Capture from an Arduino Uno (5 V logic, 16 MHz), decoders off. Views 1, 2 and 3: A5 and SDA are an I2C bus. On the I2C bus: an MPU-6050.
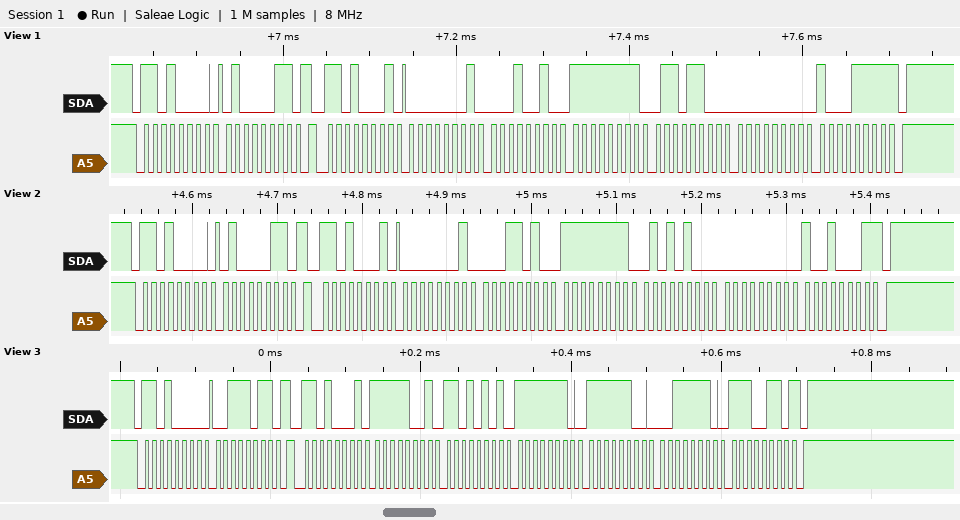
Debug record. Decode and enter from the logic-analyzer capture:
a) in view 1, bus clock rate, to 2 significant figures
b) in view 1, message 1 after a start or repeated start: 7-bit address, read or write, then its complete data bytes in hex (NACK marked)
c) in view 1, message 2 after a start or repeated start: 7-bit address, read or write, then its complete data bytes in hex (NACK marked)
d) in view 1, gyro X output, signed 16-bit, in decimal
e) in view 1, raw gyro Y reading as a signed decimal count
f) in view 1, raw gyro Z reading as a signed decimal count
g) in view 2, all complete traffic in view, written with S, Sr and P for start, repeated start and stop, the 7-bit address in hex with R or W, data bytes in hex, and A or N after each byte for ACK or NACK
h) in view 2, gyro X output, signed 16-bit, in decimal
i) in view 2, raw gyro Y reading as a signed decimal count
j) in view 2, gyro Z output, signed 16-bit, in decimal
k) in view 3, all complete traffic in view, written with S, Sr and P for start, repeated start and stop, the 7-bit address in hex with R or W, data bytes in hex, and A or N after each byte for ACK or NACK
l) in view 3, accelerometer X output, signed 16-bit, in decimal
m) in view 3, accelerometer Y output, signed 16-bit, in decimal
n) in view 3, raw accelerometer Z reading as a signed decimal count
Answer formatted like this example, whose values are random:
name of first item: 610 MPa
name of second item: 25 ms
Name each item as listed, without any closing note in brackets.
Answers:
in view 1, bus clock rate, to 2 significant figures: 100 kHz
in view 1, message 1 after a start or repeated start: 7-bit address, read or write, then its complete data bytes in hex: 0x68 write: 43
in view 1, message 2 after a start or repeated start: 7-bit address, read or write, then its complete data bytes in hex: 0x68 read: 01 12 FF 6C 00 8F NACK
in view 1, gyro X output, signed 16-bit, in decimal: 274
in view 1, raw gyro Y reading as a signed decimal count: -148
in view 1, raw gyro Z reading as a signed decimal count: 143
in view 2, all complete traffic in view, written with S, Sr and P for start, repeated start and stop, the 7-bit address in hex with R or W, data bytes in hex, and A or N after each byte for ACK or NACK: S 68W A 43 A Sr 68R A 01 A 1A A FF A 54 A 00 A 91 N P
in view 2, gyro X output, signed 16-bit, in decimal: 282
in view 2, raw gyro Y reading as a signed decimal count: -172
in view 2, gyro Z output, signed 16-bit, in decimal: 145
in view 3, all complete traffic in view, written with S, Sr and P for start, repeated start and stop, the 7-bit address in hex with R or W, data bytes in hex, and A or N after each byte for ACK or NACK: S 68W A 3B A Sr 68R A F9 A D5 A FE A FC A 3E A E6 N P
in view 3, accelerometer X output, signed 16-bit, in decimal: -1579
in view 3, accelerometer Y output, signed 16-bit, in decimal: -260
in view 3, raw accelerometer Z reading as a signed decimal count: 16102
